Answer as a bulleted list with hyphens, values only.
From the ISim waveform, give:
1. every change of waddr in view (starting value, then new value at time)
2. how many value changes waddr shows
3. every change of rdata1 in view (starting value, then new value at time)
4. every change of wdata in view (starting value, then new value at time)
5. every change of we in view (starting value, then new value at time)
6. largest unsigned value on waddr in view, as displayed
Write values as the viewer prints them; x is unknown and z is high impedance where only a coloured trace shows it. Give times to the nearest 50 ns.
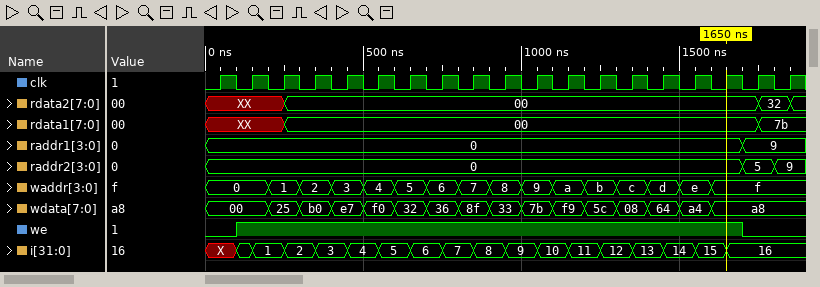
- 0, 1 at 200 ns, 2 at 300 ns, 3 at 400 ns, 4 at 500 ns, 5 at 600 ns, 6 at 700 ns, 7 at 800 ns, 8 at 900 ns, 9 at 1000 ns, a at 1100 ns, b at 1200 ns, c at 1300 ns, d at 1400 ns, e at 1500 ns, f at 1600 ns
- 15
- XX, 00 at 250 ns, 7b at 1750 ns
- 00, 25 at 200 ns, b0 at 300 ns, e7 at 400 ns, f0 at 500 ns, 32 at 600 ns, 36 at 700 ns, 8f at 800 ns, 33 at 900 ns, 7b at 1000 ns, f9 at 1100 ns, 5c at 1200 ns, 08 at 1300 ns, 64 at 1400 ns, a4 at 1500 ns, a8 at 1600 ns
- 0, 1 at 100 ns, 0 at 1700 ns
- f
